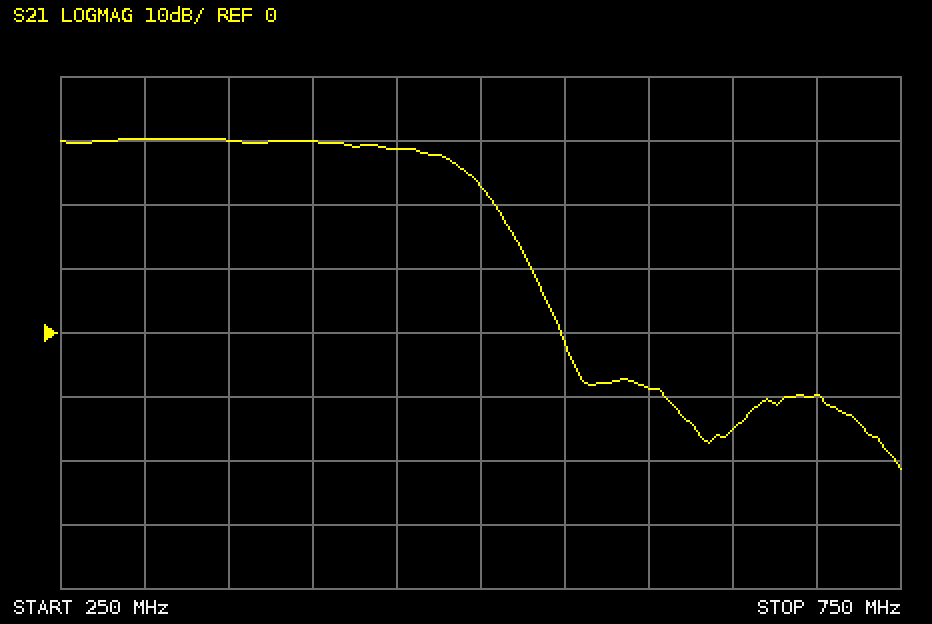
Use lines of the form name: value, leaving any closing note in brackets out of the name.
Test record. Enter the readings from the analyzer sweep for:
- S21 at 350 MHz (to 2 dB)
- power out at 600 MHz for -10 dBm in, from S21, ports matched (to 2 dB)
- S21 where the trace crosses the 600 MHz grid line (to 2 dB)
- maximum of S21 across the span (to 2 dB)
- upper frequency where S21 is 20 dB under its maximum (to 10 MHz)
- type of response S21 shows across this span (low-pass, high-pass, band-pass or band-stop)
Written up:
S21 at 350 MHz: 30 dB
power out at 600 MHz for -10 dBm in, from S21, ports matched: -18 dBm
S21 where the trace crosses the 600 MHz grid line: -8 dB
maximum of S21 across the span: 30 dB
upper frequency where S21 is 20 dB under its maximum: 530 MHz
type of response S21 shows across this span: low-pass
